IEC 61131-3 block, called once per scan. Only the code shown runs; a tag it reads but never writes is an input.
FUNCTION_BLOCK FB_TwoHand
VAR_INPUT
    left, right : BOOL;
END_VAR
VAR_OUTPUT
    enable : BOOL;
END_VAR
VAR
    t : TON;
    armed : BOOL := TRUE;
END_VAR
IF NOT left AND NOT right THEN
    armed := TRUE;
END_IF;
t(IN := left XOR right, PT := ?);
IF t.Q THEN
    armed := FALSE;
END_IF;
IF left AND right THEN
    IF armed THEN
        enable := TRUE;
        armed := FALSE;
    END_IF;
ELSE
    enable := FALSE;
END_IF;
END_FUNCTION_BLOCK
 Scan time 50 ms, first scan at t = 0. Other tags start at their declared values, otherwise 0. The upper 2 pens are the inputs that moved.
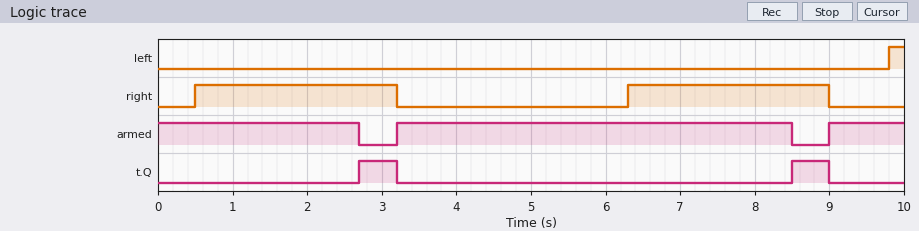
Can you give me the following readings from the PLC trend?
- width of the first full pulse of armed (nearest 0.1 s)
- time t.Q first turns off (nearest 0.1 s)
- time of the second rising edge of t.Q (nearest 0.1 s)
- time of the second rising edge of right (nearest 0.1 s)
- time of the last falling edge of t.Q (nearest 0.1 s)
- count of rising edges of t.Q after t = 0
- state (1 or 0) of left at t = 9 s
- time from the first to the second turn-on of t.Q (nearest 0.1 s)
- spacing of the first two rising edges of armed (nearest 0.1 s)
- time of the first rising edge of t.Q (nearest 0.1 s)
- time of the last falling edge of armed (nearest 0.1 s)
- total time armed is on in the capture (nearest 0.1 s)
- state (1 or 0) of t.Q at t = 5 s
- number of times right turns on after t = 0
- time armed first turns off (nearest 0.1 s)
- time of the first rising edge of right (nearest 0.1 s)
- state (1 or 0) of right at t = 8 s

5.3 s
3.2 s
8.5 s
6.3 s
9.0 s
2
0
5.8 s
5.8 s
2.7 s
8.5 s
9.0 s
0
2
2.7 s
0.5 s
1
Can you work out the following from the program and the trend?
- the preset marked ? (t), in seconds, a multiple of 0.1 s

2.2 s
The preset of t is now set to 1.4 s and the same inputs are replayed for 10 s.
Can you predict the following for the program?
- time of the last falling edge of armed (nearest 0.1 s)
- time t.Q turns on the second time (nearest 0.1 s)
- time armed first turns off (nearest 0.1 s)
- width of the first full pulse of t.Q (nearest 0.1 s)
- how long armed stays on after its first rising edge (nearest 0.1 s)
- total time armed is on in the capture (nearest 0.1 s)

7.7 s
7.7 s
1.9 s
1.3 s
4.5 s
7.4 s
